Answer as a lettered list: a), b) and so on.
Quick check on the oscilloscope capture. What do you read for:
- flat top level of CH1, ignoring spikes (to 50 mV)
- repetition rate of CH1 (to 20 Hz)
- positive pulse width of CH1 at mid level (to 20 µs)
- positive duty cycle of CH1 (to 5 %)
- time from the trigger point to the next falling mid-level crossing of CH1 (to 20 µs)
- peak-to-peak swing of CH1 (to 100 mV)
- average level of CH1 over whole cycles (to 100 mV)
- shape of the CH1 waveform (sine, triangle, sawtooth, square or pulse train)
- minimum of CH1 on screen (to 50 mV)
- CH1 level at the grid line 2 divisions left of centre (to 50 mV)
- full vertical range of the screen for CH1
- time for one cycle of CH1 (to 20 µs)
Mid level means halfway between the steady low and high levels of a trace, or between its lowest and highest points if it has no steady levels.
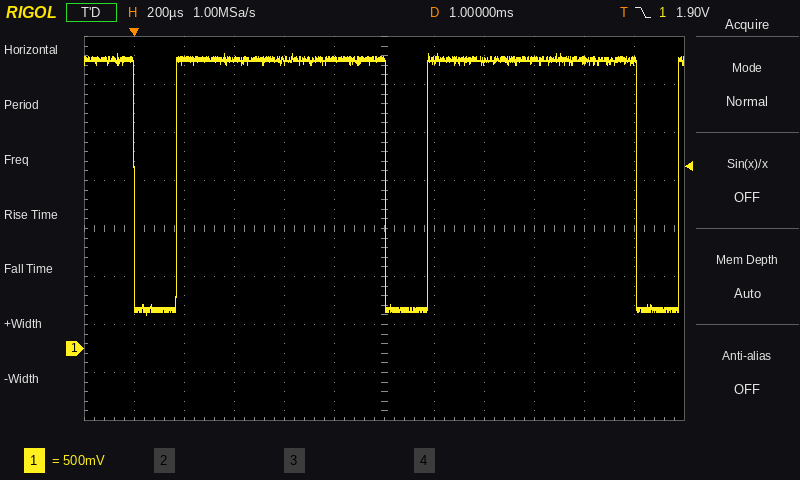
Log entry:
a) 3.00 V
b) 1.00 kHz
c) 840 µs
d) 85 %
e) 1.00 ms
f) 2.70 V
g) 2.6 V
h) pulse train
i) 350 mV
j) 3.00 V
k) 4 V
l) 1.00 ms
